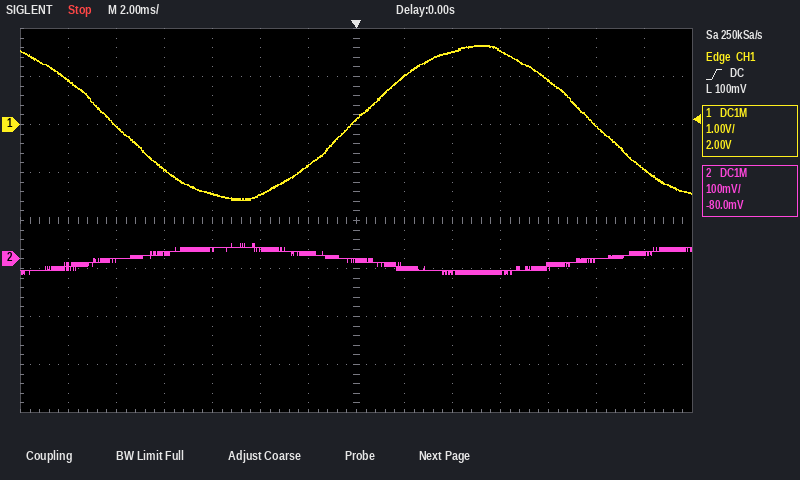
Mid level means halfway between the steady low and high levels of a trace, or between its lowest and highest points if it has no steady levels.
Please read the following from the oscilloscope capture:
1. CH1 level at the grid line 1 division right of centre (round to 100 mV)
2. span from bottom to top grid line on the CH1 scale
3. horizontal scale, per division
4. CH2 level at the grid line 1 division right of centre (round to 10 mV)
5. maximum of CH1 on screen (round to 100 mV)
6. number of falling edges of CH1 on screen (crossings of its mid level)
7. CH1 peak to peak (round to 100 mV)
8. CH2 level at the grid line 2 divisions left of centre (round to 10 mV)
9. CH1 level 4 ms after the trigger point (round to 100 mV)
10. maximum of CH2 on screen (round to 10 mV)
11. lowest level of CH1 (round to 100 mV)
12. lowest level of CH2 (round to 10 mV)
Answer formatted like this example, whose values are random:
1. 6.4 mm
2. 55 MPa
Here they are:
1. 1.0 V
2. 8 V
3. 2 ms
4. -20 mV
5. 1.6 V
6. 2
7. 3.2 V
8. 20 mV
9. 1.5 V
10. 30 mV
11. -1.6 V
12. -30 mV
